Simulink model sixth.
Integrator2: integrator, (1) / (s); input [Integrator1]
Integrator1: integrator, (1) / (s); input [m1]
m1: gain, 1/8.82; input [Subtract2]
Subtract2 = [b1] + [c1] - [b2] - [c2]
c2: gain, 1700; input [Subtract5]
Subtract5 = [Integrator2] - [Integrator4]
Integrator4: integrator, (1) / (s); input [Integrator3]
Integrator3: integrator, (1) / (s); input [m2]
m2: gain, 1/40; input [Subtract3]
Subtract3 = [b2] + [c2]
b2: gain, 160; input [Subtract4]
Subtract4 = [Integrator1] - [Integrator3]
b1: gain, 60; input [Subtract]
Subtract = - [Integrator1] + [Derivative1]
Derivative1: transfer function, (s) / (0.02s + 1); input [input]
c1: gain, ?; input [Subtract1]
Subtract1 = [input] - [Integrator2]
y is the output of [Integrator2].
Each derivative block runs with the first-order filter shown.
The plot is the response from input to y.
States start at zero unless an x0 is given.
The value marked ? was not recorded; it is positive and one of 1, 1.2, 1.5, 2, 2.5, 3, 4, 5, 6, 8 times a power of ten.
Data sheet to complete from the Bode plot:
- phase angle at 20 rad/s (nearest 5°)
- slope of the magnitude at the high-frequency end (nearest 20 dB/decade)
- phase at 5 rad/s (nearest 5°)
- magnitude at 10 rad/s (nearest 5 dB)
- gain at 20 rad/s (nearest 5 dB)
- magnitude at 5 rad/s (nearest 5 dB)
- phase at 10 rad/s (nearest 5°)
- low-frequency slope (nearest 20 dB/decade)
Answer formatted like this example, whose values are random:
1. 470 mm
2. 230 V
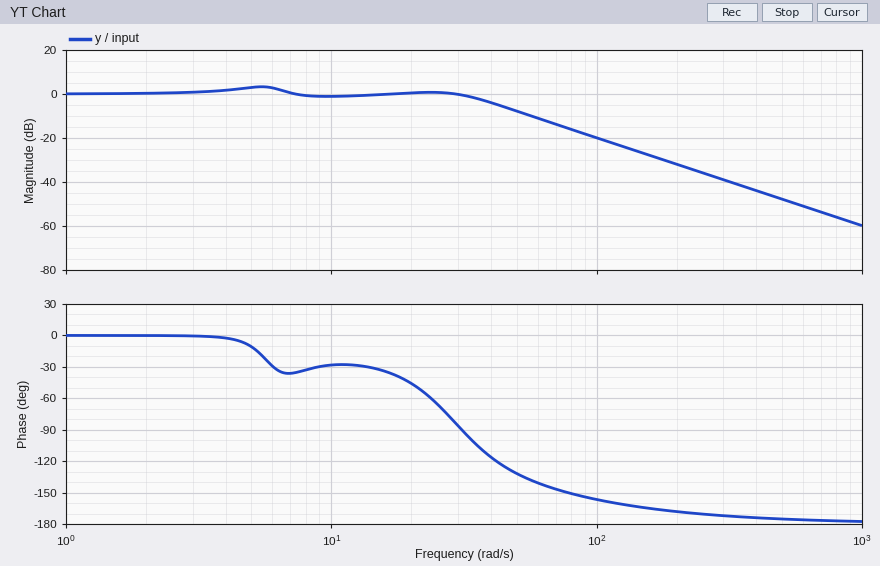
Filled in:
1. -45°
2. -40 dB/decade
3. -10°
4. 0 dB
5. 0 dB
6. 5 dB
7. -30°
8. 0 dB/decade
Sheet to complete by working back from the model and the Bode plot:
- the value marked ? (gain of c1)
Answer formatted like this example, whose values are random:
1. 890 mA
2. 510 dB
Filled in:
1. 6000
